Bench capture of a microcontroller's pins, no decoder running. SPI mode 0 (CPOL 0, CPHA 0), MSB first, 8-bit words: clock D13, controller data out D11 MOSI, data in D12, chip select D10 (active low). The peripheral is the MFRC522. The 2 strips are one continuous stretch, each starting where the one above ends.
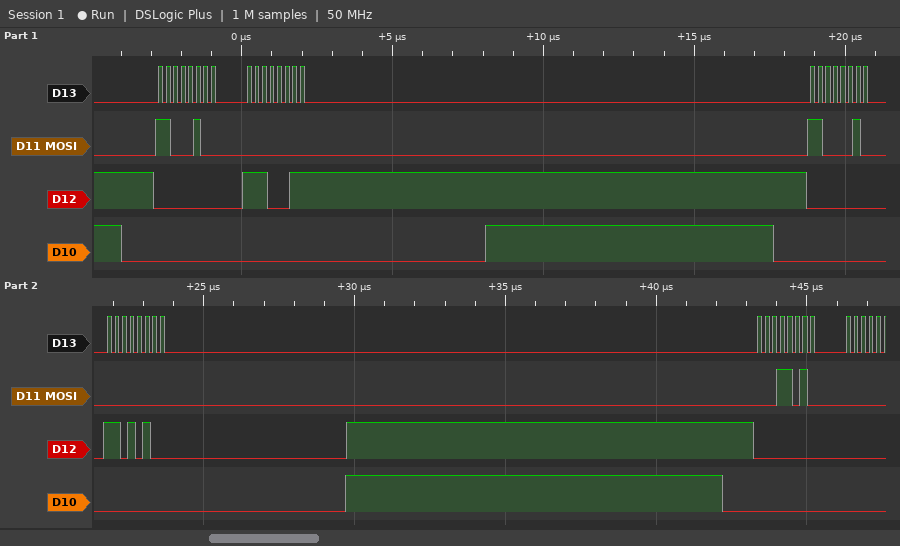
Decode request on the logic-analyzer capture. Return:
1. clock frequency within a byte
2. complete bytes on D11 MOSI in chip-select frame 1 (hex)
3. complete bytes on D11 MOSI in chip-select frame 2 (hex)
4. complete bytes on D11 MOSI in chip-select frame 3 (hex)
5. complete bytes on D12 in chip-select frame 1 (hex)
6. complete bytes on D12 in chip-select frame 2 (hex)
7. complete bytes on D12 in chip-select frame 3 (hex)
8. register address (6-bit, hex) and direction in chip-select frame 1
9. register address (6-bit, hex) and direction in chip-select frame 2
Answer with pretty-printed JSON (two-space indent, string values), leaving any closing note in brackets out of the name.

{
  "clock frequency within a byte": "4 MHz",
  "complete bytes on D11 MOSI in chip-select frame 1": "0xC4 0x00",
  "complete bytes on D11 MOSI in chip-select frame 2": "0xC2 0x00",
  "complete bytes on D11 MOSI in chip-select frame 3": "0x1A",
  "complete bytes on D12 in chip-select frame 1": "0x00 0xE3",
  "complete bytes on D12 in chip-select frame 2": "0x00 0xD4",
  "complete bytes on D12 in chip-select frame 3": "0x00",
  "register address (6-bit, hex) and direction in chip-select frame 1": "0x22 read",
  "register address (6-bit, hex) and direction in chip-select frame 2": "0x21 read"
}
